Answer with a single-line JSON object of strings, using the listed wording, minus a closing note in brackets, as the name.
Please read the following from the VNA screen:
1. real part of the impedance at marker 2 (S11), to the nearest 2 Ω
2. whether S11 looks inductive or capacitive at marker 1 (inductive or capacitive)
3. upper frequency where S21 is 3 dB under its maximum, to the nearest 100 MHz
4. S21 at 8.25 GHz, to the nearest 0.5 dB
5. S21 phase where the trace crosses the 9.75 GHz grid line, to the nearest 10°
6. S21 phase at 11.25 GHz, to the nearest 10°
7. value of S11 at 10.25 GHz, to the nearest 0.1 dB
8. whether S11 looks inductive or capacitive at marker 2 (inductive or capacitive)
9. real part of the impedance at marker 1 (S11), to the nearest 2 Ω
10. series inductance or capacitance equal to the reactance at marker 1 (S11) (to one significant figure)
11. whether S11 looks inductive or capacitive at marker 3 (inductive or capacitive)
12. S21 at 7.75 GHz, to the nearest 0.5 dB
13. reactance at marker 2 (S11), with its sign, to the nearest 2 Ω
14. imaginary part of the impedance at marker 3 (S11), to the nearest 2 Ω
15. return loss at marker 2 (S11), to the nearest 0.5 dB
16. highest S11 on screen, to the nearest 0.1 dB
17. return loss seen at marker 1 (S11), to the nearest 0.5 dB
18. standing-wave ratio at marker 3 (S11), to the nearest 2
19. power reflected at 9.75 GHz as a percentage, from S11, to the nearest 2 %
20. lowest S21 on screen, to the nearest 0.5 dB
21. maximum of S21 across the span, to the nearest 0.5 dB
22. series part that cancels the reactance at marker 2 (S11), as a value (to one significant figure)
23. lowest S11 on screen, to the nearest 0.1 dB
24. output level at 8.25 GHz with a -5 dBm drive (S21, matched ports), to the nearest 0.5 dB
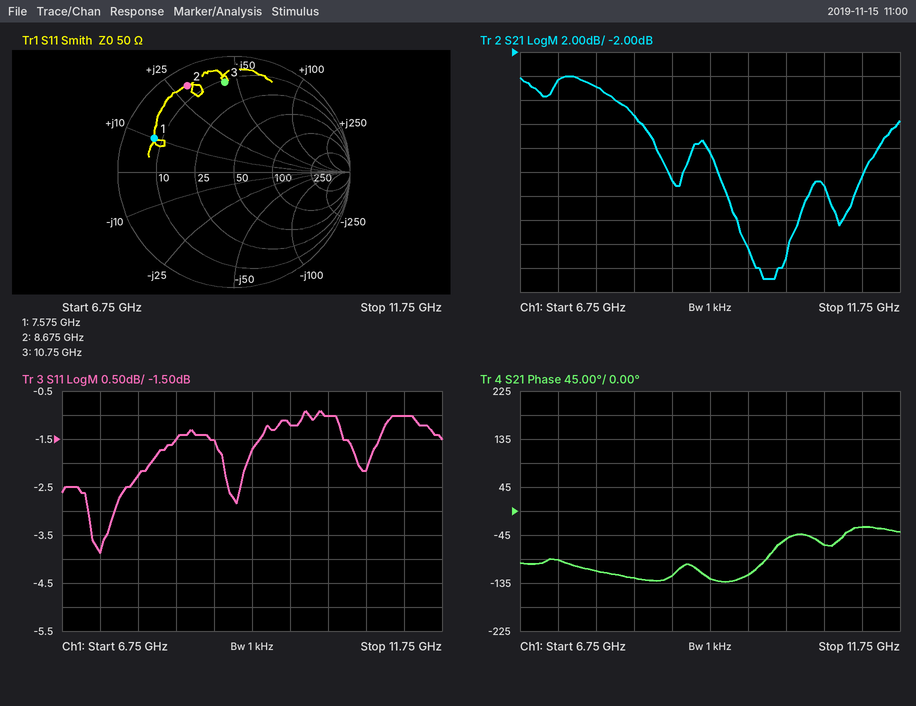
{"real part of the impedance at marker 2 (S11), to the nearest 2 Ω": "6 Ω", "whether S11 looks inductive or capacitive at marker 1": "inductive", "upper frequency where S21 is 3 dB under its maximum, to the nearest 100 MHz": "8.2 GHz", "S21 at 8.25 GHz, to the nearest 0.5 dB": "-7.5 dB", "S21 phase where the trace crosses the 9.75 GHz grid line, to the nearest 10°": "-120°", "S21 phase at 11.25 GHz, to the nearest 10°": "-30°", "value of S11 at 10.25 GHz, to the nearest 0.1 dB": "-1.0 dB", "whether S11 looks inductive or capacitive at marker 2": "inductive", "real part of the impedance at marker 1 (S11), to the nearest 2 Ω": "8 Ω", "series inductance or capacitance equal to the reactance at marker 1 (S11)": "200 pH", "whether S11 looks inductive or capacitive at marker 3": "inductive", "S21 at 7.75 GHz, to the nearest 0.5 dB": "-5.0 dB", "reactance at marker 2 (S11), with its sign, to the nearest 2 Ω": "+30 Ω", "imaginary part of the impedance at marker 3 (S11), to the nearest 2 Ω": "+44 Ω", "return loss at marker 2 (S11), to the nearest 0.5 dB": "1.5 dB", "highest S11 on screen, to the nearest 0.1 dB": "-0.9 dB", "return loss seen at marker 1 (S11), to the nearest 0.5 dB": "2.5 dB", "standing-wave ratio at marker 3 (S11), to the nearest 2": "8", "power reflected at 9.75 GHz as a percentage, from S11, to the nearest 2 %": "76 %", "lowest S21 on screen, to the nearest 0.5 dB": "-21.0 dB", "maximum of S21 across the span, to the nearest 0.5 dB": "-4.0 dB", "series part that cancels the reactance at marker 2 (S11), as a value": "600 fF", "lowest S11 on screen, to the nearest 0.1 dB": "-3.9 dB", "output level at 8.25 GHz with a -5 dBm drive (S21, matched ports), to the nearest 0.5 dB": "-12.5 dBm"}
